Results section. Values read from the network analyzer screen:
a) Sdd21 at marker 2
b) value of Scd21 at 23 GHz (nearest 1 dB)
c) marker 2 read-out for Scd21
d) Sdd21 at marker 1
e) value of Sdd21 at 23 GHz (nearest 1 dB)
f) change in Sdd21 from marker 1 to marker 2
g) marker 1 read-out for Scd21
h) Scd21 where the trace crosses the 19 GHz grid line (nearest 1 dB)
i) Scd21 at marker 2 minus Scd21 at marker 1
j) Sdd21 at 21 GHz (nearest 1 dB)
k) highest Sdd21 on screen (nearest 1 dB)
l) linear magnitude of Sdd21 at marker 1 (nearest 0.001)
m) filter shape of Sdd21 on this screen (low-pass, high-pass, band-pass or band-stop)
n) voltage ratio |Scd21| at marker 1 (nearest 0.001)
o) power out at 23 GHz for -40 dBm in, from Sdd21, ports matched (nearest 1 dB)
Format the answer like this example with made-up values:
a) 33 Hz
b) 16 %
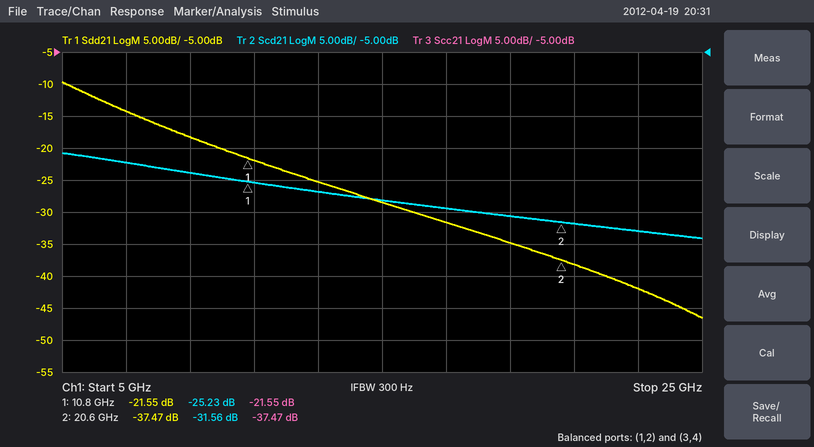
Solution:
a) -37.47 dB
b) -33 dB
c) -31.56 dB
d) -21.55 dB
e) -42 dB
f) -15.92 dB
g) -25.23 dB
h) -31 dB
i) -6.33 dB
j) -38 dB
k) -10 dB
l) 0.084
m) low-pass
n) 0.055
o) -82 dBm
